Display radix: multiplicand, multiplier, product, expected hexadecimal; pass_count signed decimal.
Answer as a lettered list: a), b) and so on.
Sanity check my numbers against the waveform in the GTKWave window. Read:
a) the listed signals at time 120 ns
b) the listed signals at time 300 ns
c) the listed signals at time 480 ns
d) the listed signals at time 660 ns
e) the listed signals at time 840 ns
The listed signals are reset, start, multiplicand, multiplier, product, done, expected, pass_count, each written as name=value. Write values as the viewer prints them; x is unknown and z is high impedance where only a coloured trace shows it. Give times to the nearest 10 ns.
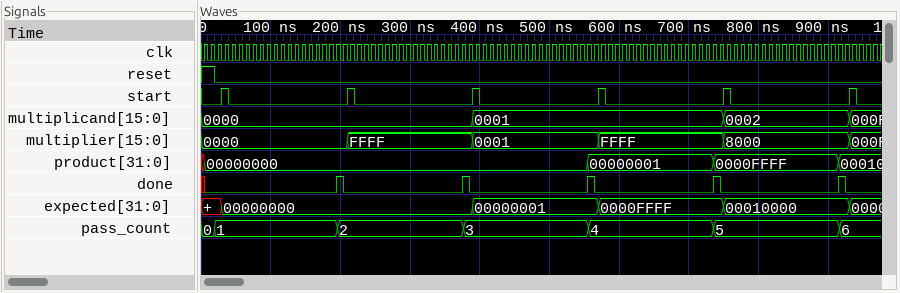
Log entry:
a) reset=0, start=0, multiplicand=0000, multiplier=0000, product=00000000, done=0, expected=00000000, pass_count=1
b) reset=0, start=0, multiplicand=0000, multiplier=FFFF, product=00000000, done=0, expected=00000000, pass_count=2
c) reset=0, start=0, multiplicand=0001, multiplier=0001, product=00000000, done=0, expected=00000001, pass_count=3
d) reset=0, start=0, multiplicand=0001, multiplier=FFFF, product=00000001, done=0, expected=0000FFFF, pass_count=4
e) reset=0, start=0, multiplicand=0002, multiplier=8000, product=0000FFFF, done=0, expected=00010000, pass_count=5
